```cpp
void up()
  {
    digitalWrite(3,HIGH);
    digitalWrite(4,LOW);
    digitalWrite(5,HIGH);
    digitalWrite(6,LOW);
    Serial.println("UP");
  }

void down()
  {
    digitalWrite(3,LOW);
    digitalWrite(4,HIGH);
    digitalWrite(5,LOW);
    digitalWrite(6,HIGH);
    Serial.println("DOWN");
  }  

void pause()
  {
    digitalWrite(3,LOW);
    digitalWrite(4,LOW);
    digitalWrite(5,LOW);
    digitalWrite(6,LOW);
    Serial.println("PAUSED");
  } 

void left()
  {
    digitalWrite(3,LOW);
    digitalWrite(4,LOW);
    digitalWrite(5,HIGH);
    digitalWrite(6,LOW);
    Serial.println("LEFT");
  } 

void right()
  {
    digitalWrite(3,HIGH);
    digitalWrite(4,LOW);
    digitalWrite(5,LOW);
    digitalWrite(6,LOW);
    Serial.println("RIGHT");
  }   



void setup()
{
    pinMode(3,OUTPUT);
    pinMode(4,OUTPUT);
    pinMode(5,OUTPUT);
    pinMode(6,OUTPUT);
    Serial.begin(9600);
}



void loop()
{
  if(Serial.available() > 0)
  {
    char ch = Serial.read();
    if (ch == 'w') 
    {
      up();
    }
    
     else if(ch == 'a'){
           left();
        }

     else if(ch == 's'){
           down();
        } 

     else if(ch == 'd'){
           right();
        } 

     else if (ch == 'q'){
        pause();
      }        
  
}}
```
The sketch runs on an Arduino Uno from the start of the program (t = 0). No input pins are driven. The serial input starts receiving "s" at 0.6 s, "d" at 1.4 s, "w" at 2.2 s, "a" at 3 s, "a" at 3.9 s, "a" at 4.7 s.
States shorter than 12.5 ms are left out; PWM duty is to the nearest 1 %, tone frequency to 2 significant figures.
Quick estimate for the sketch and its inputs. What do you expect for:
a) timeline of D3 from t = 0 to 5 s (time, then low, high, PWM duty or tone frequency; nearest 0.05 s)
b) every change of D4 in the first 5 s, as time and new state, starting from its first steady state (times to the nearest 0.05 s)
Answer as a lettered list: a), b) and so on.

a) 0 s low; 1.4 s high; 3 s low
b) 0 s low; 0.6 s high; 1.4 s low
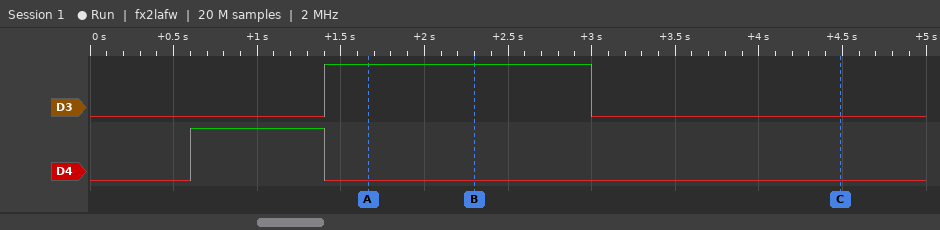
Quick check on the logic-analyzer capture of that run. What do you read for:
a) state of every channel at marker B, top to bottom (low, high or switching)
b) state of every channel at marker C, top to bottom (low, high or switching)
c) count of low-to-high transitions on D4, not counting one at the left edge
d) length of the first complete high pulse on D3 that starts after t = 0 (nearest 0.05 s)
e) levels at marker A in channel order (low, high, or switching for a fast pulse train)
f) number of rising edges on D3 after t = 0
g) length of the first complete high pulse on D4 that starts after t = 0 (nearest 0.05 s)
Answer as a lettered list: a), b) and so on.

a) D3 high, D4 low
b) D3 low, D4 low
c) 1
d) 1.60 s
e) D3 high, D4 low
f) 1
g) 0.80 s
